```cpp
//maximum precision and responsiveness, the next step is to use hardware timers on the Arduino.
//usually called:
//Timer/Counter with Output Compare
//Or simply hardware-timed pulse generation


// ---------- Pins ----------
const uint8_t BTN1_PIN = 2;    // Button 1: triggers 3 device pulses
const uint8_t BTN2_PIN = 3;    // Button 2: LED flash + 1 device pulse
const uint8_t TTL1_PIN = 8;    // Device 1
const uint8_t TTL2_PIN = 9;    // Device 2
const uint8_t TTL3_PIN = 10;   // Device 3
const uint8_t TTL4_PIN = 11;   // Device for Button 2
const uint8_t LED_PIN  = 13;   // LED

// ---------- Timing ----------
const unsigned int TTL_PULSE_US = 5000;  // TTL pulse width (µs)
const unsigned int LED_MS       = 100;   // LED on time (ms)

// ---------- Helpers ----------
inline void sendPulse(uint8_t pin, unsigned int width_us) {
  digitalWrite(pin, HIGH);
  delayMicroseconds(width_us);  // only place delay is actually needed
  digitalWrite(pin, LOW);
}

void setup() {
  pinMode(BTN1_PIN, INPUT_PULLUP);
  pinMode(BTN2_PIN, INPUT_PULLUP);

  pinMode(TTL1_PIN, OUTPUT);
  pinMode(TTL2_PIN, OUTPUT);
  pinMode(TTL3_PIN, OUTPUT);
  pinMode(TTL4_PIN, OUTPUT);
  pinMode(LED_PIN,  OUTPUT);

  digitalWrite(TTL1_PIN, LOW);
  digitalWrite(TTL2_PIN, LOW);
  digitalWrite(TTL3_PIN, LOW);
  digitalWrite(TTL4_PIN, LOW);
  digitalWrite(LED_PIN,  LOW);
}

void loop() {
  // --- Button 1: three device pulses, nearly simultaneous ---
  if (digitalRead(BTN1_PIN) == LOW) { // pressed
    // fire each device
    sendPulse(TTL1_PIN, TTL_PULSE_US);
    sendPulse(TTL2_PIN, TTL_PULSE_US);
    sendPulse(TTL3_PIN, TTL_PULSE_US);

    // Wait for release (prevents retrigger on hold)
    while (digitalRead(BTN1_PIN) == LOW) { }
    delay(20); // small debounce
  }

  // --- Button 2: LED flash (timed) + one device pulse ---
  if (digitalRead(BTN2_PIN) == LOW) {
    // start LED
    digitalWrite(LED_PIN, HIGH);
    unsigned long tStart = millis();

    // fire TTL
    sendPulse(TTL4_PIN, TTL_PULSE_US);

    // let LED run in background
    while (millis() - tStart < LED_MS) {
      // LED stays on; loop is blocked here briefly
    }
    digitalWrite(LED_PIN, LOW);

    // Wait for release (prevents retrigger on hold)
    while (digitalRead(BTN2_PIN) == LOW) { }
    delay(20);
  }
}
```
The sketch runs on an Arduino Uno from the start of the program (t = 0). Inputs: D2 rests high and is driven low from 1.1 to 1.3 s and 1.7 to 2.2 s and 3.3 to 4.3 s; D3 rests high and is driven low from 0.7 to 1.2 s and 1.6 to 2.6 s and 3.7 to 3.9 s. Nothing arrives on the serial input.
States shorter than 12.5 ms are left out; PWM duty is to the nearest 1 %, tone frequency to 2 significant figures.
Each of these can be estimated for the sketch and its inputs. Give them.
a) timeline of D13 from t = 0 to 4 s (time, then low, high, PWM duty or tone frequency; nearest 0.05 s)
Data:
0 s low; 0.7 s high; 0.8 s low; 1.6 s high; 1.7 s low
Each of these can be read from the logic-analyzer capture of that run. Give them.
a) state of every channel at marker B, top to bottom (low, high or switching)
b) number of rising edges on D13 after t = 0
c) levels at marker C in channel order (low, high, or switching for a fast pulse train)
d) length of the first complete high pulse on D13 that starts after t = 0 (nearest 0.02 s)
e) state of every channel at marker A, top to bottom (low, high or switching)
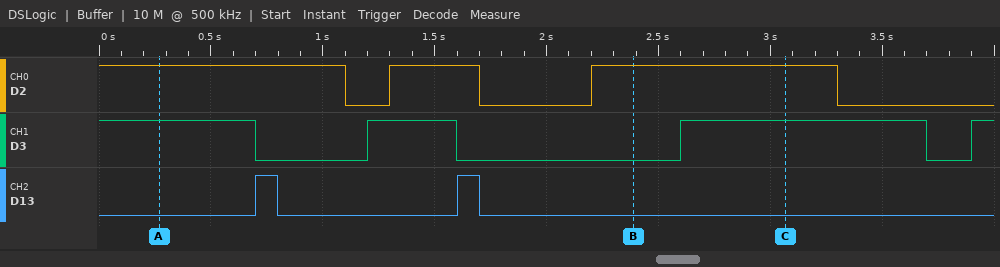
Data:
D2 high, D3 low, D13 low
2
D2 high, D3 high, D13 low
0.10 s
D2 high, D3 high, D13 low
